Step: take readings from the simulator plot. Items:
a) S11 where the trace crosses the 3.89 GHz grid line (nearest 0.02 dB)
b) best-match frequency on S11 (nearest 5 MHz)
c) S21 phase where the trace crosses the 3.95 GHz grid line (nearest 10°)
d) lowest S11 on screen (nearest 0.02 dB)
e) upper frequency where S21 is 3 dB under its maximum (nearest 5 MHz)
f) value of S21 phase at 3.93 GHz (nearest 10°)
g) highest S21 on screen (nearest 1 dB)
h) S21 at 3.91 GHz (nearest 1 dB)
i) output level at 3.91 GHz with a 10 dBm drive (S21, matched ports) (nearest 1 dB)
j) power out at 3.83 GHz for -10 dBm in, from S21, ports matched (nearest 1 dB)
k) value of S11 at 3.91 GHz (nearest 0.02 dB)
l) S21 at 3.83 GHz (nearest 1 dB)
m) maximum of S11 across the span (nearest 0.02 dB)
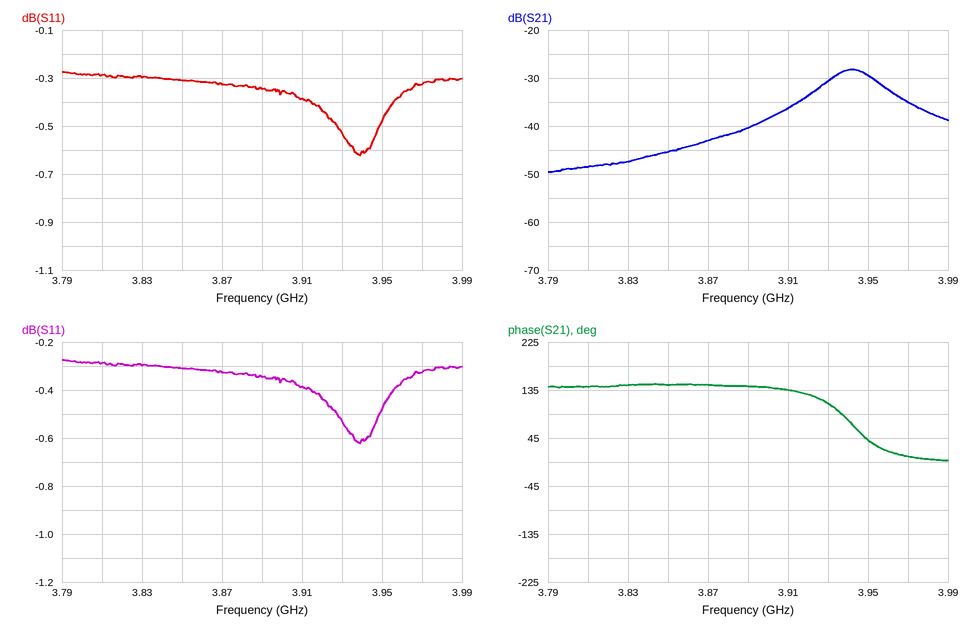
-0.34 dB
3.940 GHz
40°
-0.62 dB
3.955 GHz
110°
-28 dB
-36 dB
-26 dBm
-57 dBm
-0.38 dB
-47 dB
-0.28 dB
